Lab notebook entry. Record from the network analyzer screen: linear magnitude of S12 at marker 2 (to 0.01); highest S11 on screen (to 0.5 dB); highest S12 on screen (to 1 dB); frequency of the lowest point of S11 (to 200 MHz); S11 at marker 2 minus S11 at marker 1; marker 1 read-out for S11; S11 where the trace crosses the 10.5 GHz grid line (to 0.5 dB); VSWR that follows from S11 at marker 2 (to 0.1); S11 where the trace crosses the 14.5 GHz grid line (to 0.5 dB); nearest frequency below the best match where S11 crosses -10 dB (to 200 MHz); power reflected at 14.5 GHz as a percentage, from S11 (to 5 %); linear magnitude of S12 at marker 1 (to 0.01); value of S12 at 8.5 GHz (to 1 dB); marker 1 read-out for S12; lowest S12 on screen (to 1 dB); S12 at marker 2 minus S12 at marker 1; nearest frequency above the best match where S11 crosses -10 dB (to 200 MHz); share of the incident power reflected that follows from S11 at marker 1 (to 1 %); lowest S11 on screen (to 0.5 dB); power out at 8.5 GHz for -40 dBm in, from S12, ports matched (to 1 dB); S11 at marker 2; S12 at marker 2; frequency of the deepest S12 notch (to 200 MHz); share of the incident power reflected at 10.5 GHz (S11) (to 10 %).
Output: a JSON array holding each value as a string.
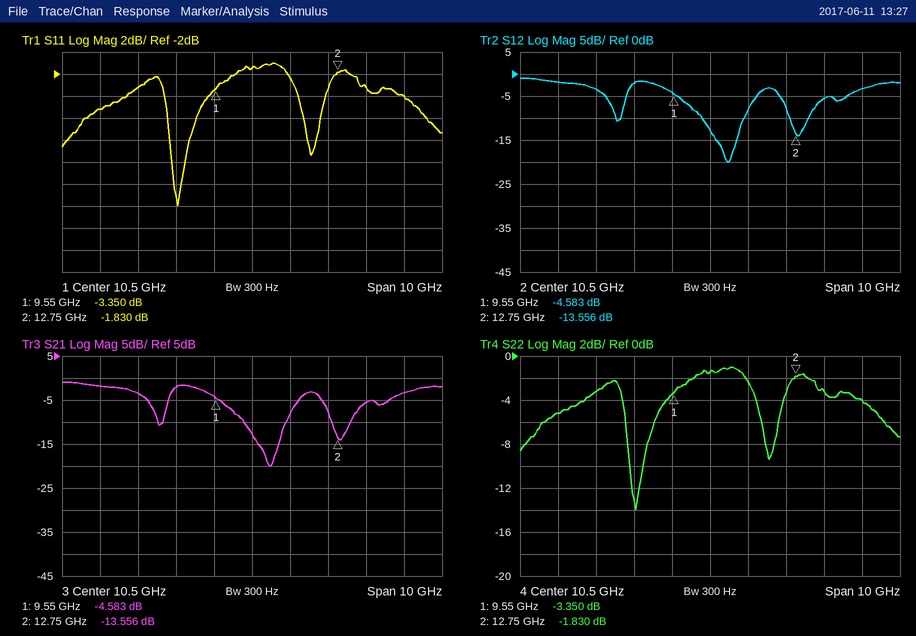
["0.21", "-1.0 dB", "-1 dB", "8.6 GHz", "1.520 dB", "-3.350 dB", "-1.5 dB", "9.5", "-4.0 dB", "8.4 GHz", "40 %", "0.59", "-2 dB", "-4.583 dB", "-20 dB", "-8.973 dB", "8.8 GHz", "46 %", "-14.0 dB", "-42 dBm", "-1.830 dB", "-13.556 dB", "11.0 GHz", "70 %"]
